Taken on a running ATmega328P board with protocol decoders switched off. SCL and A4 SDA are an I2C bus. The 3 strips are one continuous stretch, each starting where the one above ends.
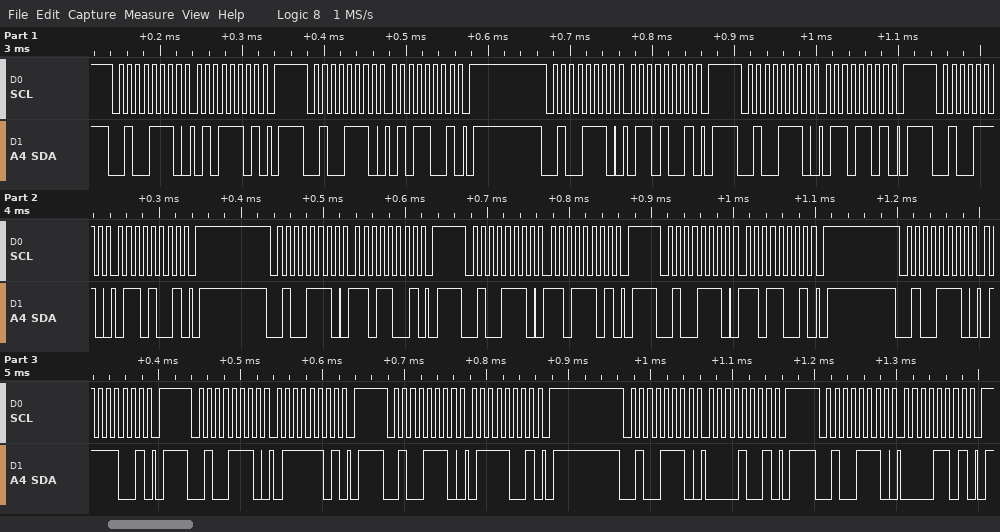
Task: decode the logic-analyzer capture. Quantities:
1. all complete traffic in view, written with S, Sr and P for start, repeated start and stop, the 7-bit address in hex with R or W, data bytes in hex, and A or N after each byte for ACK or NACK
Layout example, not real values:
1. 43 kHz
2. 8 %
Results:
1. S 27W A 5D A P S 27W A 59 A P S 27W A 69 A P S 27W A 6D A P S 27W A 69 A P S 27W A D9 A P S 27W A DD A P S 27W A D9 A P S 27W A 79 A P S 27W A 7D A P S 27W A 79 A P S 27W A 09 A P S 27W A 0D A P
